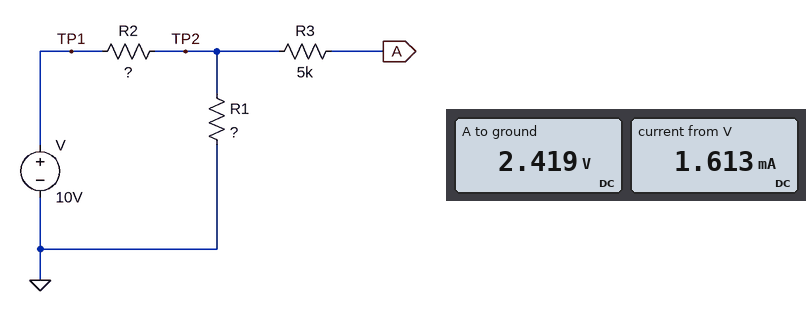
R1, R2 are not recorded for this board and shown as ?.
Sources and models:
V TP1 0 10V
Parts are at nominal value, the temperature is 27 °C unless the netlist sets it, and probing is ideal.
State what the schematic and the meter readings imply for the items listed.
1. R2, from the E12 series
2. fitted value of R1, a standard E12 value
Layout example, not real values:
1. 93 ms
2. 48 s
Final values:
1. 4.7 kΩ
2. 1.5 kΩ
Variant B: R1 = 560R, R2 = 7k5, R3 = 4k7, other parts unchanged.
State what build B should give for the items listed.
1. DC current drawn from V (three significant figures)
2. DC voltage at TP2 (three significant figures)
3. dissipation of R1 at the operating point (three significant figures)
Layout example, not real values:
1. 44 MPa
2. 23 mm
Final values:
1. 1.24 mA
2. 695 mV
3. 862 µW
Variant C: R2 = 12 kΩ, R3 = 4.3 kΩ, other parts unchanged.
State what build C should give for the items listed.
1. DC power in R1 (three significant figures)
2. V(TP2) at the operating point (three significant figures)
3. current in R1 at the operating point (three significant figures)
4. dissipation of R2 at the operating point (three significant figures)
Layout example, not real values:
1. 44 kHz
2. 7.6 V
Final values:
1. 823 µW
2. 1.11 V
3. 741 µA
4. 6.58 mW
